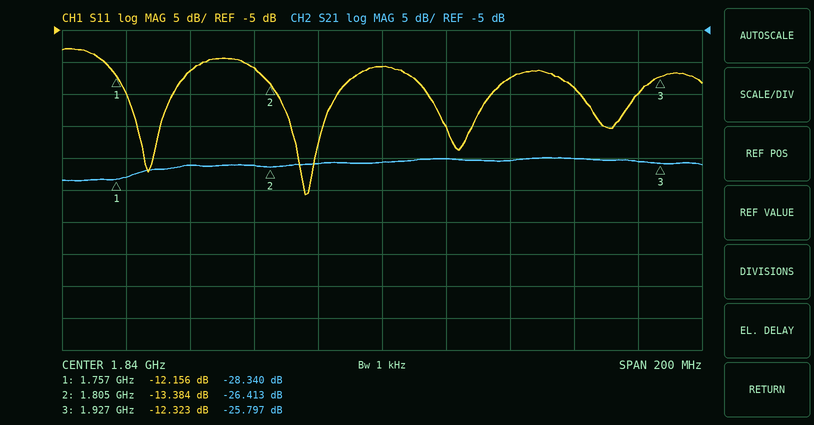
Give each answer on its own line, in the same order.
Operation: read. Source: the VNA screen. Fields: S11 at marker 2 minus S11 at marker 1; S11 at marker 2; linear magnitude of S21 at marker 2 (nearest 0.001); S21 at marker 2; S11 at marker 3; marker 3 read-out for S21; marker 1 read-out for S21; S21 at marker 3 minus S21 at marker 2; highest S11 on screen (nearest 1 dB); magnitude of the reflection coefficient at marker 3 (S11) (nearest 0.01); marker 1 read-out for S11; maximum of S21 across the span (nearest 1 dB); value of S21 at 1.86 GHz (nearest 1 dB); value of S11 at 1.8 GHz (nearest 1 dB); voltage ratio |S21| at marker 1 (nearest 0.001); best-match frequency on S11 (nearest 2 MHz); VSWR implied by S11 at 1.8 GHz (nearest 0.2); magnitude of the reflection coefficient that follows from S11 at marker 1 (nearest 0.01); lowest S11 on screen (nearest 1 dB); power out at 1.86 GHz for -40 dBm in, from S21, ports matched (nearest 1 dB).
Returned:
-1.228 dB
-13.384 dB
0.048
-26.413 dB
-12.323 dB
-25.797 dB
-28.340 dB
0.616 dB
-8 dB
0.24
-12.156 dB
-25 dB
-25 dB
-11 dB
0.038
1.816 GHz
1.8
0.25
-31 dB
-65 dBm
